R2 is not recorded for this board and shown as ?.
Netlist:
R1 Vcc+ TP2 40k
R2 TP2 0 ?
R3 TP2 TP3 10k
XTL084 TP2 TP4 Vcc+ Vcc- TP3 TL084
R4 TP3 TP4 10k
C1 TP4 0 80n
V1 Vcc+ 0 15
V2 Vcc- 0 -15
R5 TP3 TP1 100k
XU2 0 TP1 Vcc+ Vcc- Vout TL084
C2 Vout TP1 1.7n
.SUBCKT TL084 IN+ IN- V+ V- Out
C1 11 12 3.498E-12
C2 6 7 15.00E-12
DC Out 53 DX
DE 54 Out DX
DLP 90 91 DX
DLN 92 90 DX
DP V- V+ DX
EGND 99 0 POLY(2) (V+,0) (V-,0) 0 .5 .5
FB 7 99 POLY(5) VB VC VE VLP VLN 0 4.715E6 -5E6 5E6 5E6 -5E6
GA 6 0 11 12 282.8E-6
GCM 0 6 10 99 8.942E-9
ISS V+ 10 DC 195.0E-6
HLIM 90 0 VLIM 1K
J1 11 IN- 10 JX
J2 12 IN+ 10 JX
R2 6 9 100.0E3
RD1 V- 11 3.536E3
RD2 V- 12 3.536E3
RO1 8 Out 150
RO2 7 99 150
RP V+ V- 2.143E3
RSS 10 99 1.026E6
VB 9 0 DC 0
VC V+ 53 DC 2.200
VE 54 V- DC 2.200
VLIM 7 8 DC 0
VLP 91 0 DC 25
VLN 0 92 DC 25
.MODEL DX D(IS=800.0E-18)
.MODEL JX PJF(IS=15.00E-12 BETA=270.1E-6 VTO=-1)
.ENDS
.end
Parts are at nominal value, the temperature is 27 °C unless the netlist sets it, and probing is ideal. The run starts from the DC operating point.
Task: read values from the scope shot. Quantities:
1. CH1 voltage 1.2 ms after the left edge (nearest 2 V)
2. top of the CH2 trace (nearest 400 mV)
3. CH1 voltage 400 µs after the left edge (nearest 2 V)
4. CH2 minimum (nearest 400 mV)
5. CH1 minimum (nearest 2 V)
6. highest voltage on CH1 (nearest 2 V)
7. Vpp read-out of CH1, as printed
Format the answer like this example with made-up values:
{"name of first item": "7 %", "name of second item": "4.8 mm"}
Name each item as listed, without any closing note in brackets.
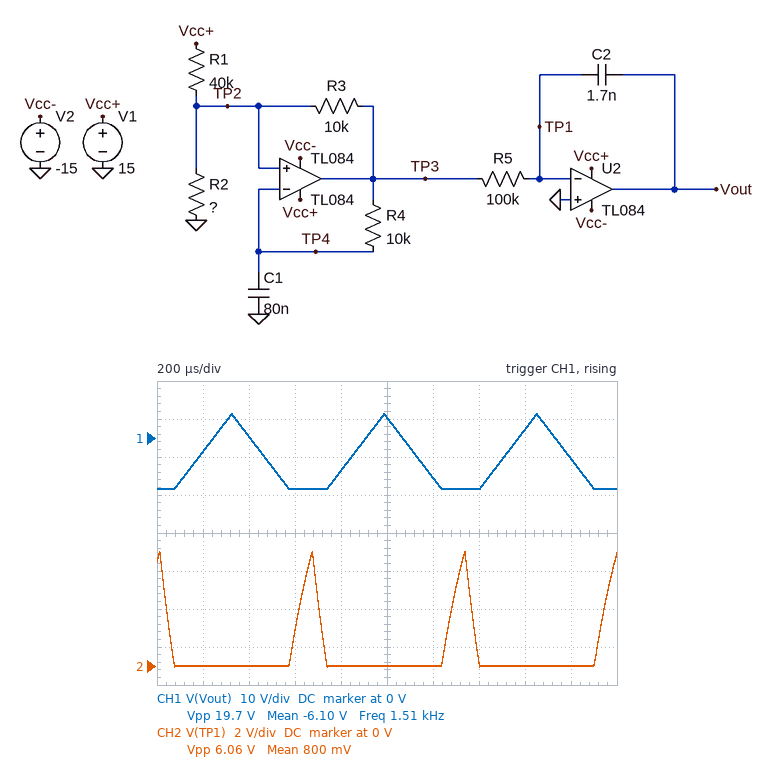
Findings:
{"CH1 voltage 1.2 ms after the left edge": "-10 V", "top of the CH2 trace": "6.0 V", "CH1 voltage 400 µs after the left edge": "0 V", "CH2 minimum": "0 V", "CH1 minimum": "-14 V", "highest voltage on CH1": "6 V", "Vpp read-out of CH1, as printed": "19.7 V"}
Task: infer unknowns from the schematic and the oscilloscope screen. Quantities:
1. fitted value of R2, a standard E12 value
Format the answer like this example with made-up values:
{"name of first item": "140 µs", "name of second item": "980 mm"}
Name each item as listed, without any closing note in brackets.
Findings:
{"fitted value of R2, a standard E12 value": "2.7 kΩ"}
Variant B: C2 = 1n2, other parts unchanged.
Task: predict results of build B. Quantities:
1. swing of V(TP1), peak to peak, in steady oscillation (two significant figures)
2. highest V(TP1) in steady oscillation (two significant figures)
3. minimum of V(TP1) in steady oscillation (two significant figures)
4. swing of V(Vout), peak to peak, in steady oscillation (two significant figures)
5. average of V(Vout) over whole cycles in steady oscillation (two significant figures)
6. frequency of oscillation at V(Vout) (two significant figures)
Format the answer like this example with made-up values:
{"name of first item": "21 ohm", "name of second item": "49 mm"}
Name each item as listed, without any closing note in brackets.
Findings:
{"swing of V(TP1), peak to peak, in steady oscillation": "9.3 V", "highest V(TP1) in steady oscillation": "7.2 V", "minimum of V(TP1) in steady oscillation": "-2.1 V", "swing of V(Vout), peak to peak, in steady oscillation": "27 V", "average of V(Vout) over whole cycles in steady oscillation": "-2.2 V", "frequency of oscillation at V(Vout)": "1.5 kHz"}
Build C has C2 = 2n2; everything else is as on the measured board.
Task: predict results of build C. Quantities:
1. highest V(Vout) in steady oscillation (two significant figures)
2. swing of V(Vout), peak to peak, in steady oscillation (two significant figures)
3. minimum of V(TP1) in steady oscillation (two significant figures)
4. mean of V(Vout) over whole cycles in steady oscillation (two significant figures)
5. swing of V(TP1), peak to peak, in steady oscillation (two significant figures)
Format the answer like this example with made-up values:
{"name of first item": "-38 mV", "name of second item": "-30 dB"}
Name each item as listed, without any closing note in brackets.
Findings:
{"highest V(Vout) in steady oscillation": "1.1 V", "swing of V(Vout), peak to peak, in steady oscillation": "15 V", "minimum of V(TP1) in steady oscillation": "-42 mV", "mean of V(Vout) over whole cycles in steady oscillation": "-8.2 V", "swing of V(TP1), peak to peak, in steady oscillation": "5.4 V"}
